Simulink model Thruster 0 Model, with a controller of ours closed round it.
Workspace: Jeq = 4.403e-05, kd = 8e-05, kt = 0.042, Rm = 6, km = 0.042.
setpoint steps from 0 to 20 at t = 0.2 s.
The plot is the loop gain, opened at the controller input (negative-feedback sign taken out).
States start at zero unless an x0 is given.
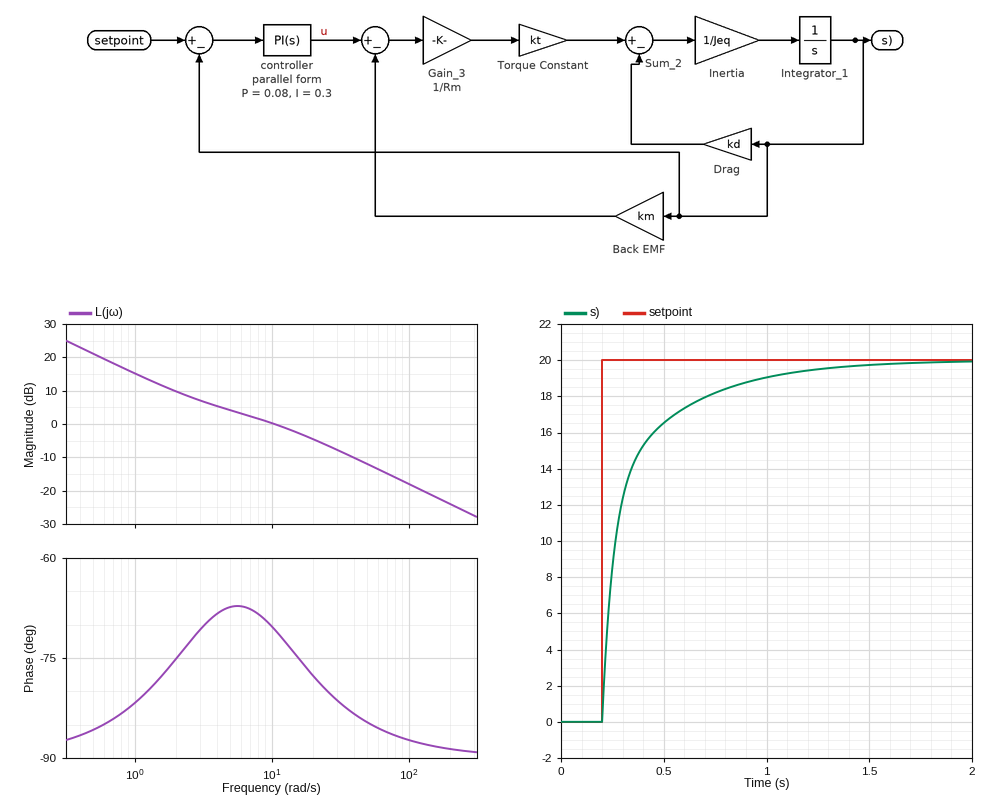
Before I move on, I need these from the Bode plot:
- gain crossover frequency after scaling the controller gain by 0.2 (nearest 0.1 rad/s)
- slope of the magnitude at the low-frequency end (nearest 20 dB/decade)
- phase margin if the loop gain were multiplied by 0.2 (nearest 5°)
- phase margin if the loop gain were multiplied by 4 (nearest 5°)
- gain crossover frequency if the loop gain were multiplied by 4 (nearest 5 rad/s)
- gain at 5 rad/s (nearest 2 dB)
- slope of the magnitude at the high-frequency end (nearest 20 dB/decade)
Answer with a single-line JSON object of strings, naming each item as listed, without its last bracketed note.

{"gain crossover frequency after scaling the controller gain by 0.2": "1.2 rad/s", "slope of the magnitude at the low-frequency end": "-20 dB/decade", "phase margin if the loop gain were multiplied by 0.2": "100°", "phase margin if the loop gain were multiplied by 4": "95°", "gain crossover frequency if the loop gain were multiplied by 4": "50 rad/s", "gain at 5 rad/s": "4 dB", "slope of the magnitude at the high-frequency end": "-20 dB/decade"}
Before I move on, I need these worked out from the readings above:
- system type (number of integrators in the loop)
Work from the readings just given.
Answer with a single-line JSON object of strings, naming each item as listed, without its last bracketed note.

{"system type": "1"}
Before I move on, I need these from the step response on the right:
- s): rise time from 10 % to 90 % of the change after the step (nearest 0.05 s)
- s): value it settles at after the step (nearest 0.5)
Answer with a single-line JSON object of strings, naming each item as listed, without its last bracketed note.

{"s): rise time from 10 % to 90 % of the change after the step": "0.50 s", "s): value it settles at after the step": "20.0"}
